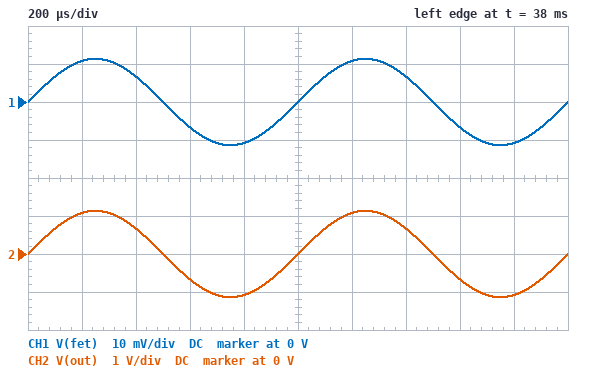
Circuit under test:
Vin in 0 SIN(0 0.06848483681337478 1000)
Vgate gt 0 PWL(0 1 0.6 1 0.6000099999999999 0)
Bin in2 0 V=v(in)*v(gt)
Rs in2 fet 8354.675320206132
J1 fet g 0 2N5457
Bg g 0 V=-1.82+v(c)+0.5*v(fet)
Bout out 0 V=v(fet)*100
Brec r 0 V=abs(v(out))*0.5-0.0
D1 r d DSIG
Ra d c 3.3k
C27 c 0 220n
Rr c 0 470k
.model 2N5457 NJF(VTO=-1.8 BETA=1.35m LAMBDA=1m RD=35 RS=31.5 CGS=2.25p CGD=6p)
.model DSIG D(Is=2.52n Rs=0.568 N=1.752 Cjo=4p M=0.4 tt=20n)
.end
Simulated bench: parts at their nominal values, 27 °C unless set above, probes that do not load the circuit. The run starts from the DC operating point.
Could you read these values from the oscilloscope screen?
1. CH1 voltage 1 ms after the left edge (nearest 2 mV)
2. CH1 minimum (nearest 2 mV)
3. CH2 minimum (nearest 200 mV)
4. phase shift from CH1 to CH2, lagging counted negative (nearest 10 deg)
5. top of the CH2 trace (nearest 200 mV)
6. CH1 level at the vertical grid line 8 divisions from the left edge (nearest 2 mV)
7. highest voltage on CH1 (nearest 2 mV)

0 V
-12 mV
-1.2 V
0 deg
1.2 V
-6 mV
12 mV
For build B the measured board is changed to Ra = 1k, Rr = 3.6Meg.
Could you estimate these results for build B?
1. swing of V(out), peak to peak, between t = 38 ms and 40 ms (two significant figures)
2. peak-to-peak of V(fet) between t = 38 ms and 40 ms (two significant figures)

2.1 V
21 mV
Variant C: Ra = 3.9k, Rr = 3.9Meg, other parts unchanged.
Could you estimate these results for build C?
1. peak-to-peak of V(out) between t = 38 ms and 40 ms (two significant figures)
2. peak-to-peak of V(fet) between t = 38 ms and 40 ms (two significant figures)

2.1 V
21 mV
